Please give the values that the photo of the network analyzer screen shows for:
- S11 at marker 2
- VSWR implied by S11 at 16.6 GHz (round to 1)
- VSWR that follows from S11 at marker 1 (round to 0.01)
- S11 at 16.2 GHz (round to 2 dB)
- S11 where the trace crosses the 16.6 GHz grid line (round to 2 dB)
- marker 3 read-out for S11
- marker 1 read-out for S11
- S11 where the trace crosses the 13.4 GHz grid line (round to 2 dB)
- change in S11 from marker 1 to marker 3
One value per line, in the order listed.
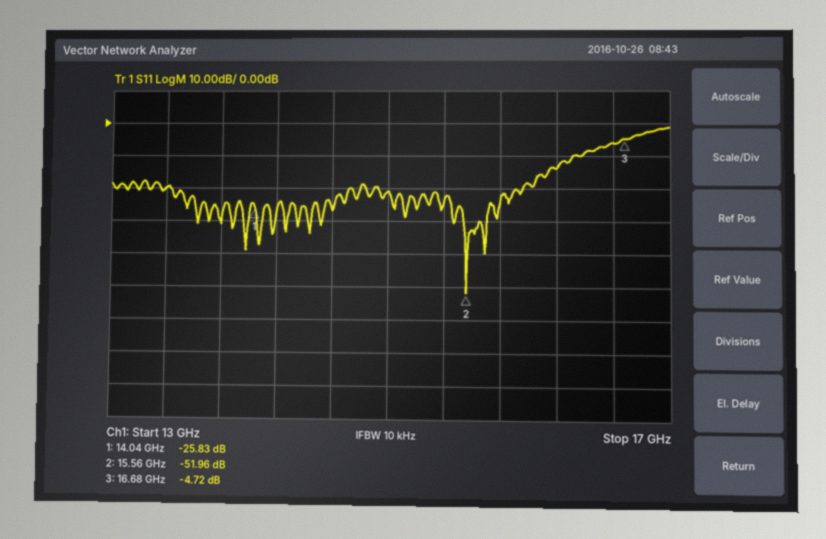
-51.96 dB
3
1.11
-14 dB
-6 dB
-4.72 dB
-25.83 dB
-20 dB
21.11 dB
